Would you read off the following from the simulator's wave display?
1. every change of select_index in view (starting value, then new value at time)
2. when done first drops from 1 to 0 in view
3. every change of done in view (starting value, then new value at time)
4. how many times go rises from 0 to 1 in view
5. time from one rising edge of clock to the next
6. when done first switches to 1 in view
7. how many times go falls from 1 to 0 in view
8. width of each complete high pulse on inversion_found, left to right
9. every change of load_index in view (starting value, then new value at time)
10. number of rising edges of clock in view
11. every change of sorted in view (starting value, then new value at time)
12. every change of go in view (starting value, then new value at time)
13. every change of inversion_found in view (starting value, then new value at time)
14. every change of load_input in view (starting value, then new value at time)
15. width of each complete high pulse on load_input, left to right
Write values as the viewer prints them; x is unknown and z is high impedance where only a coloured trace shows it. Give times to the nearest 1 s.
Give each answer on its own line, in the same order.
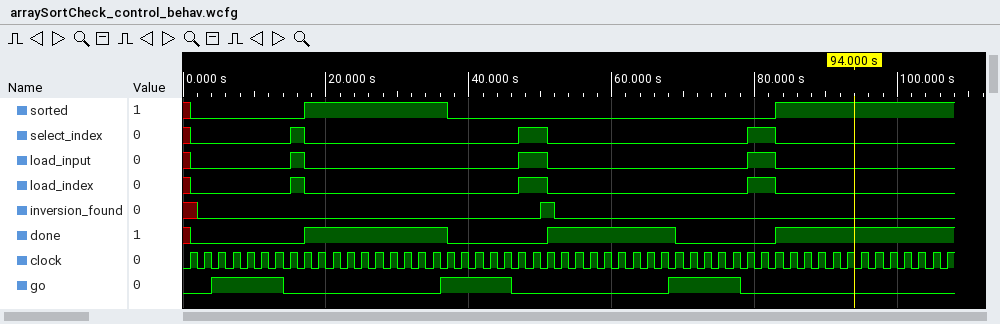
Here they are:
x, 0 at 1 s, 1 at 15 s, 0 at 17 s, 1 at 47 s, 0 at 51 s, 1 at 79 s, 0 at 83 s
37 s
x, 0 at 1 s, 1 at 17 s, 0 at 37 s, 1 at 51 s, 0 at 69 s, 1 at 83 s
3
2 s
17 s
3
2 s
x, 0 at 1 s, 1 at 15 s, 0 at 17 s, 1 at 47 s, 0 at 51 s, 1 at 79 s, 0 at 83 s
54
x, 0 at 1 s, 1 at 17 s, 0 at 37 s, 1 at 83 s
0, 1 at 4 s, 0 at 14 s, 1 at 36 s, 0 at 46 s, 1 at 68 s, 0 at 78 s
x, 0 at 2 s, 1 at 50 s, 0 at 52 s
x, 0 at 1 s, 1 at 15 s, 0 at 17 s, 1 at 47 s, 0 at 51 s, 1 at 79 s, 0 at 83 s
2 s, 4 s, 4 s
